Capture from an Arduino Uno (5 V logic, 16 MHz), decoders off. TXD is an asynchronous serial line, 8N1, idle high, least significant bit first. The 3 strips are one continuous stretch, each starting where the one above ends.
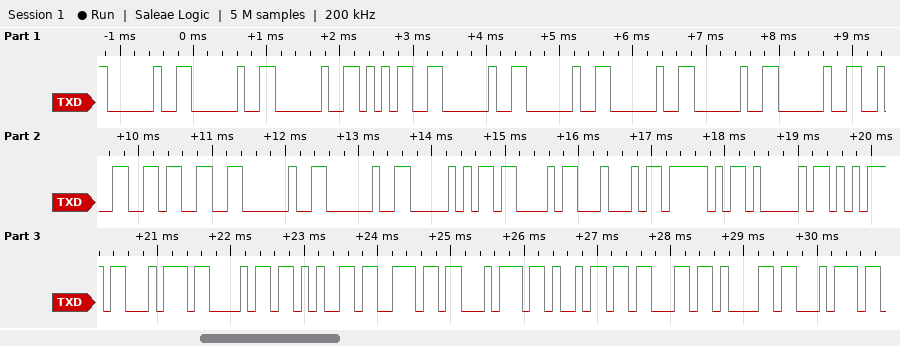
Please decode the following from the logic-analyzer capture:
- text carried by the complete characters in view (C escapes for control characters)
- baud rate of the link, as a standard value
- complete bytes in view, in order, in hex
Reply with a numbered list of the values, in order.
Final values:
1. "   5     23  PCD_Authenticat"
2. 9600 baud
3. 20 20 20 35 20 20 20 20 20 32 33 20 20 50 43 44 5F 41 75 74 68 65 6E 74 69 63 61 74
